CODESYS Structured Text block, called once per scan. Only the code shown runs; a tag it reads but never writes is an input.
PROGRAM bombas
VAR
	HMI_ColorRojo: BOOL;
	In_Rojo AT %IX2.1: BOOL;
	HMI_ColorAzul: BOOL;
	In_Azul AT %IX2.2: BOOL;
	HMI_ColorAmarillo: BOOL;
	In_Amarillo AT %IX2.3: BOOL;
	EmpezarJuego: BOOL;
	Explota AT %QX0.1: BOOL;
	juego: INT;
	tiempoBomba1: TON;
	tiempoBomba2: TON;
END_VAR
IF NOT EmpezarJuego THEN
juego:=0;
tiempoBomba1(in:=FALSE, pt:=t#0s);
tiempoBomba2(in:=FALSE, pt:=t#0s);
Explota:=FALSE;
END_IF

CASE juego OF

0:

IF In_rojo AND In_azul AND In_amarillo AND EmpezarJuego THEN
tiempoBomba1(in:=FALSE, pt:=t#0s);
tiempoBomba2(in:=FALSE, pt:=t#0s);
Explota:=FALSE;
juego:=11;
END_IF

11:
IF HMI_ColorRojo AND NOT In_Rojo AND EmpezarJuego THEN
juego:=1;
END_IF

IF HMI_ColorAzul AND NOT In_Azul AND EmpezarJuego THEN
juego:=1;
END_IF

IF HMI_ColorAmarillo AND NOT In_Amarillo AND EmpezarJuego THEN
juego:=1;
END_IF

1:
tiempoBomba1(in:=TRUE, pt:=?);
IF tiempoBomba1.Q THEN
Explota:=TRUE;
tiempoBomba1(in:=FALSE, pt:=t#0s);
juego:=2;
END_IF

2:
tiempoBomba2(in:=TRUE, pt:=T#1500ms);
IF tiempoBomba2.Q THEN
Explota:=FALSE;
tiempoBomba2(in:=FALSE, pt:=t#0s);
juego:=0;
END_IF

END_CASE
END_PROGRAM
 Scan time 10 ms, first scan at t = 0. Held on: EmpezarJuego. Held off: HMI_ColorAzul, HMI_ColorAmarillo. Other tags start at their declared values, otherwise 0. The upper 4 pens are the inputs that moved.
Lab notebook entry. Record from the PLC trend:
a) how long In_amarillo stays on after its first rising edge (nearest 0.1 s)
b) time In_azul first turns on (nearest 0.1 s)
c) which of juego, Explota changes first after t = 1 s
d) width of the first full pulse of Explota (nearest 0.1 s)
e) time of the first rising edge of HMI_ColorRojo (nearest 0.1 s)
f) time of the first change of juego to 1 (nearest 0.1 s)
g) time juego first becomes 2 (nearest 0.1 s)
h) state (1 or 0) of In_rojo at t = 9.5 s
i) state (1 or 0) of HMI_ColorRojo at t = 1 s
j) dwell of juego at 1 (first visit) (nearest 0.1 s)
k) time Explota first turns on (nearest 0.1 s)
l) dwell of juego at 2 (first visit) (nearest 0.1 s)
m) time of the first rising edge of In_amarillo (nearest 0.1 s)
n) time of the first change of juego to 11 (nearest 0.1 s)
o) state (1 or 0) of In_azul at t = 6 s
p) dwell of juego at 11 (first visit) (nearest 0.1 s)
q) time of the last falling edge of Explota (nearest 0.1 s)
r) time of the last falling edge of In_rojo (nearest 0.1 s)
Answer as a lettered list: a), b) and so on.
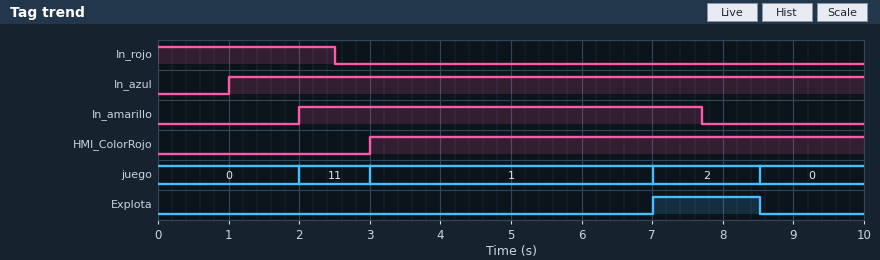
a) 5.7 s
b) 1.0 s
c) juego
d) 1.5 s
e) 3.0 s
f) 3.0 s
g) 7.0 s
h) 0
i) 0
j) 4.0 s
k) 7.0 s
l) 1.5 s
m) 2.0 s
n) 2.0 s
o) 1
p) 1.0 s
q) 8.5 s
r) 2.5 s
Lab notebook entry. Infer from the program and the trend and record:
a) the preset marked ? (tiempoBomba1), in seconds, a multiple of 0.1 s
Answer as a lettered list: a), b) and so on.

a) 4.0 s
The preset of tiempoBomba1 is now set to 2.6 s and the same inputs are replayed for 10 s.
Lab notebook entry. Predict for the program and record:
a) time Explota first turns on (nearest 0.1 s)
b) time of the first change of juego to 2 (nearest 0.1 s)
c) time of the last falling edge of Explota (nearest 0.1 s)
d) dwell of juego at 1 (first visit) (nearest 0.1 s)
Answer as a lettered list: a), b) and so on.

a) 5.6 s
b) 5.6 s
c) 7.1 s
d) 2.6 s
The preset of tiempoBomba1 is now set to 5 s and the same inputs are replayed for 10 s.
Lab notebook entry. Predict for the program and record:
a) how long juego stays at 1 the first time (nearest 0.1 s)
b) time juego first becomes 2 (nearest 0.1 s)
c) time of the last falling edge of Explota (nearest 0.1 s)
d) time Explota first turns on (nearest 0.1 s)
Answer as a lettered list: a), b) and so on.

a) 5.0 s
b) 8.0 s
c) 9.5 s
d) 8.0 s
